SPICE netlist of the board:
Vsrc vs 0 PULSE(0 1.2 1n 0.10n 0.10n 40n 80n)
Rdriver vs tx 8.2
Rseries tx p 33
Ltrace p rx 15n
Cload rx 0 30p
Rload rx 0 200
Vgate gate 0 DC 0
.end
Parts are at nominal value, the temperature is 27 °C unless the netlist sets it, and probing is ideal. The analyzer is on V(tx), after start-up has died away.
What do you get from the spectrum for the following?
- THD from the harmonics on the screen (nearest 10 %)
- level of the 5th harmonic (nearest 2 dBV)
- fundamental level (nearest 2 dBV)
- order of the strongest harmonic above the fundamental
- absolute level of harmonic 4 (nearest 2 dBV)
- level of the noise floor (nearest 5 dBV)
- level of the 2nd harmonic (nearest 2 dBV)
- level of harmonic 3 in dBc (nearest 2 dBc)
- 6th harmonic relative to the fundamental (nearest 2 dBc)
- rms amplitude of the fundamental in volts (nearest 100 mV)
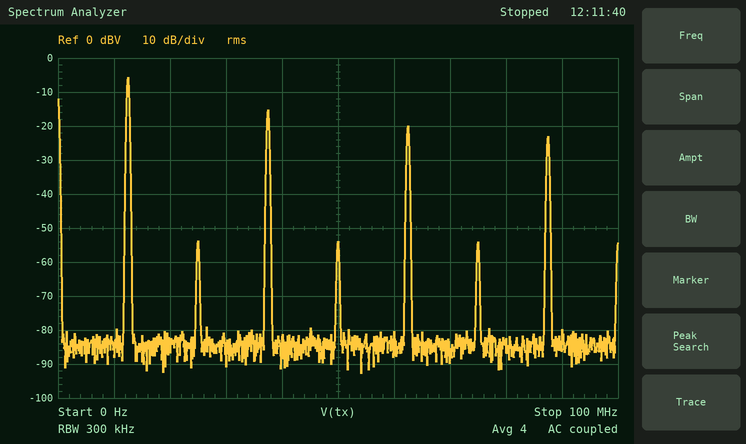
40 %
-20 dBV
-6 dBV
3
-54 dBV
-85 dBV
-54 dBV
-10 dBc
-48 dBc
500 mV
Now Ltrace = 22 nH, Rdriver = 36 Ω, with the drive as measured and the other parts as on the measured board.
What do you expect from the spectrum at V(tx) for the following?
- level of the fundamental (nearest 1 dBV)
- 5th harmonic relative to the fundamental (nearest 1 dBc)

-7 dBV
-15 dBc
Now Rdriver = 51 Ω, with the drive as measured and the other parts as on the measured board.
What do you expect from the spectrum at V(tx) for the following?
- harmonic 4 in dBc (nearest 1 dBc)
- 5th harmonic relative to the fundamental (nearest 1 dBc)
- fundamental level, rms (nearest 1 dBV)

-49 dBc
-15 dBc
-7 dBV
